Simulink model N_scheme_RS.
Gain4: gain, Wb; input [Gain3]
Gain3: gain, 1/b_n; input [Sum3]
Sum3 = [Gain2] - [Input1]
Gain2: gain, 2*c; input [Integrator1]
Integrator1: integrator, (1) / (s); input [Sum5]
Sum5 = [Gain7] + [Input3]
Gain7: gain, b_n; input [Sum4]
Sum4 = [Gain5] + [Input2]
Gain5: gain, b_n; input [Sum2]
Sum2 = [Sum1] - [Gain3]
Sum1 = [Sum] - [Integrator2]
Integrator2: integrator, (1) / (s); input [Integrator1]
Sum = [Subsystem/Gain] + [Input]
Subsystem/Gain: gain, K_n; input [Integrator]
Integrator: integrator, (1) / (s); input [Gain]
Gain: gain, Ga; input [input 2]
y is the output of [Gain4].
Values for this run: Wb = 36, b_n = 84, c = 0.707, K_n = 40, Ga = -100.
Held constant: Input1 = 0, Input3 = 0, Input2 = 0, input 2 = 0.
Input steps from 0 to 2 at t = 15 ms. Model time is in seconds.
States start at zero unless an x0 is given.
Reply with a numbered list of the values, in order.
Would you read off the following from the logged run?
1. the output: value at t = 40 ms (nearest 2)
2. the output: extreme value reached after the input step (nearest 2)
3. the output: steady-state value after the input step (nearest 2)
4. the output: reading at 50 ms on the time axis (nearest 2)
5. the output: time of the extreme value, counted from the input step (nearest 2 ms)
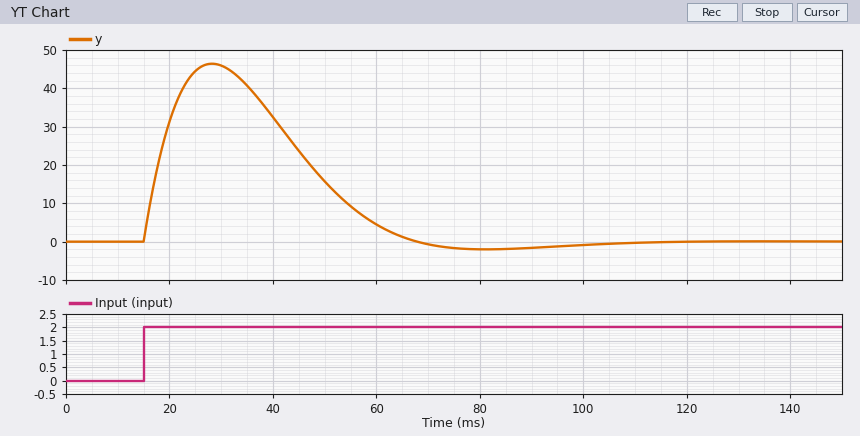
1. 32
2. 46
3. 0
4. 16
5. 14 ms
